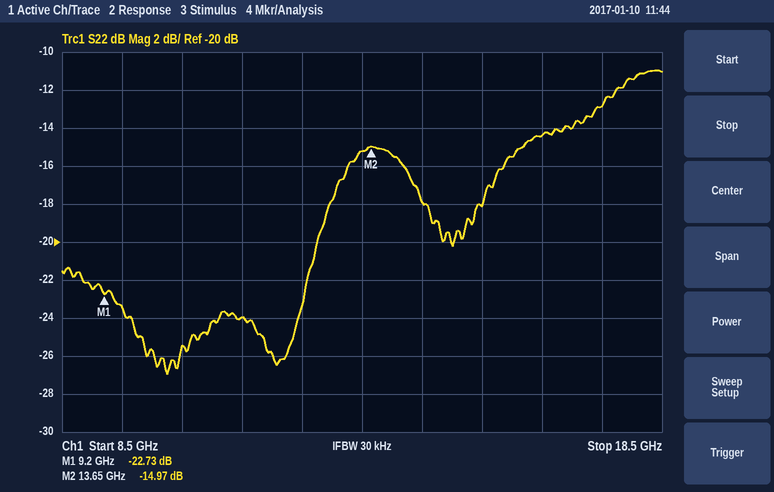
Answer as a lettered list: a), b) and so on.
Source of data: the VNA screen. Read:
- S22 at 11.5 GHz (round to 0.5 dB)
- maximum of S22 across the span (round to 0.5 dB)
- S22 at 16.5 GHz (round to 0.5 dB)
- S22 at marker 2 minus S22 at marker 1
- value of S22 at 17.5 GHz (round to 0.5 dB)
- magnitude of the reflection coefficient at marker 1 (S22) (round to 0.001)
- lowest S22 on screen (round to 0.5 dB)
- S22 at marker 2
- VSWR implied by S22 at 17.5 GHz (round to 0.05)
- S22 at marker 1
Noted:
a) -24.0 dB
b) -11.0 dB
c) -14.5 dB
d) 7.76 dB
e) -13.0 dB
f) 0.073
g) -27.0 dB
h) -14.97 dB
i) 1.60
j) -22.73 dB
